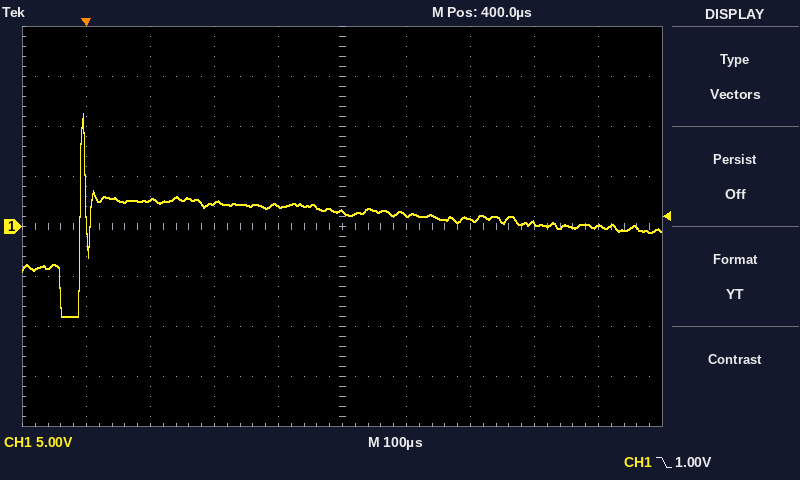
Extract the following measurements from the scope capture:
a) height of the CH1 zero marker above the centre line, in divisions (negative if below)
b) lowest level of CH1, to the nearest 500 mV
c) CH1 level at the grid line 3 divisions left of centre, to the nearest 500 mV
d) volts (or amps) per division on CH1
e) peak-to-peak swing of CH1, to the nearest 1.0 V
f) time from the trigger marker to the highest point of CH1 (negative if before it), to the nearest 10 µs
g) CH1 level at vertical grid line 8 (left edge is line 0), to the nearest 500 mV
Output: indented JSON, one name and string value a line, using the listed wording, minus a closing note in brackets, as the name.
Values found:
{
  "height of the CH1 zero marker above the centre line, in divisions": "0.0 div",
  "lowest level of CH1, to the nearest 500 mV": "-9.0 V",
  "CH1 level at the grid line 3 divisions left of centre, to the nearest 500 mV": "2.5 V",
  "volts (or amps) per division on CH1": "5 V",
  "peak-to-peak swing of CH1, to the nearest 1.0 V": "20.0 V",
  "time from the trigger marker to the highest point of CH1 (negative if before it), to the nearest 10 µs": "0 µs",
  "CH1 level at vertical grid line 8 (left edge is line 0), to the nearest 500 mV": "500 mV"
}
